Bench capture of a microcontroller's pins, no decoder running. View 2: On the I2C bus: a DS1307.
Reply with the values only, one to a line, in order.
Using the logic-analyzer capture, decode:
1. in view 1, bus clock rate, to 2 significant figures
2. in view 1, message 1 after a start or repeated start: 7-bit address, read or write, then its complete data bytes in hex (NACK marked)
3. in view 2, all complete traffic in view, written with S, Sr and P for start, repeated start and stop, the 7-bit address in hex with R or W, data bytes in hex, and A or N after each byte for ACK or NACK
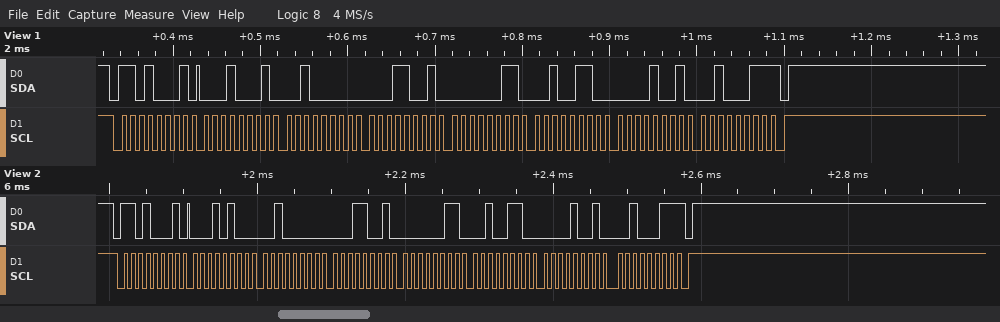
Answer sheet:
100 kHz
0x68 read: 11 20 19 03 26 09 23 NACK
S 68R A 14 A 20 A 19 A 03 A 26 A 09 A 23 N P
